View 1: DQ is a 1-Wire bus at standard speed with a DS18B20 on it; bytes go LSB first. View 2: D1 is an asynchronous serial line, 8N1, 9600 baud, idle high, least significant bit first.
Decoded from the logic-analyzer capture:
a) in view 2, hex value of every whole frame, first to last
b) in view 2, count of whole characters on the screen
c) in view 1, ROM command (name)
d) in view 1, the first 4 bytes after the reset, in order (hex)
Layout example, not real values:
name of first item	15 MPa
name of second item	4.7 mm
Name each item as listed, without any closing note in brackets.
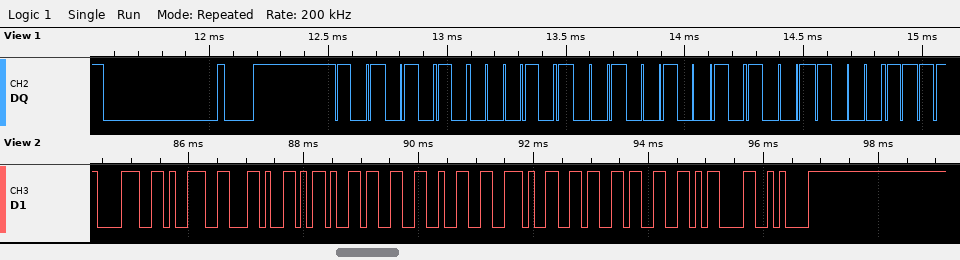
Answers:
in view 2, hex value of every whole frame, first to last	0x38 0x39 0x2C 0x2D 0x33 0x32 0x2E 0x36 0x33 0x0D 0x0A
in view 2, count of whole characters on the screen	11
in view 1, ROM command	Match ROM
in view 1, the first 4 bytes after the reset, in order	55 28 49 19
